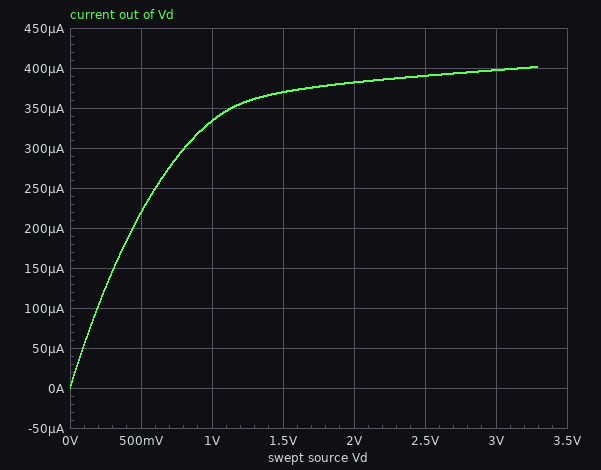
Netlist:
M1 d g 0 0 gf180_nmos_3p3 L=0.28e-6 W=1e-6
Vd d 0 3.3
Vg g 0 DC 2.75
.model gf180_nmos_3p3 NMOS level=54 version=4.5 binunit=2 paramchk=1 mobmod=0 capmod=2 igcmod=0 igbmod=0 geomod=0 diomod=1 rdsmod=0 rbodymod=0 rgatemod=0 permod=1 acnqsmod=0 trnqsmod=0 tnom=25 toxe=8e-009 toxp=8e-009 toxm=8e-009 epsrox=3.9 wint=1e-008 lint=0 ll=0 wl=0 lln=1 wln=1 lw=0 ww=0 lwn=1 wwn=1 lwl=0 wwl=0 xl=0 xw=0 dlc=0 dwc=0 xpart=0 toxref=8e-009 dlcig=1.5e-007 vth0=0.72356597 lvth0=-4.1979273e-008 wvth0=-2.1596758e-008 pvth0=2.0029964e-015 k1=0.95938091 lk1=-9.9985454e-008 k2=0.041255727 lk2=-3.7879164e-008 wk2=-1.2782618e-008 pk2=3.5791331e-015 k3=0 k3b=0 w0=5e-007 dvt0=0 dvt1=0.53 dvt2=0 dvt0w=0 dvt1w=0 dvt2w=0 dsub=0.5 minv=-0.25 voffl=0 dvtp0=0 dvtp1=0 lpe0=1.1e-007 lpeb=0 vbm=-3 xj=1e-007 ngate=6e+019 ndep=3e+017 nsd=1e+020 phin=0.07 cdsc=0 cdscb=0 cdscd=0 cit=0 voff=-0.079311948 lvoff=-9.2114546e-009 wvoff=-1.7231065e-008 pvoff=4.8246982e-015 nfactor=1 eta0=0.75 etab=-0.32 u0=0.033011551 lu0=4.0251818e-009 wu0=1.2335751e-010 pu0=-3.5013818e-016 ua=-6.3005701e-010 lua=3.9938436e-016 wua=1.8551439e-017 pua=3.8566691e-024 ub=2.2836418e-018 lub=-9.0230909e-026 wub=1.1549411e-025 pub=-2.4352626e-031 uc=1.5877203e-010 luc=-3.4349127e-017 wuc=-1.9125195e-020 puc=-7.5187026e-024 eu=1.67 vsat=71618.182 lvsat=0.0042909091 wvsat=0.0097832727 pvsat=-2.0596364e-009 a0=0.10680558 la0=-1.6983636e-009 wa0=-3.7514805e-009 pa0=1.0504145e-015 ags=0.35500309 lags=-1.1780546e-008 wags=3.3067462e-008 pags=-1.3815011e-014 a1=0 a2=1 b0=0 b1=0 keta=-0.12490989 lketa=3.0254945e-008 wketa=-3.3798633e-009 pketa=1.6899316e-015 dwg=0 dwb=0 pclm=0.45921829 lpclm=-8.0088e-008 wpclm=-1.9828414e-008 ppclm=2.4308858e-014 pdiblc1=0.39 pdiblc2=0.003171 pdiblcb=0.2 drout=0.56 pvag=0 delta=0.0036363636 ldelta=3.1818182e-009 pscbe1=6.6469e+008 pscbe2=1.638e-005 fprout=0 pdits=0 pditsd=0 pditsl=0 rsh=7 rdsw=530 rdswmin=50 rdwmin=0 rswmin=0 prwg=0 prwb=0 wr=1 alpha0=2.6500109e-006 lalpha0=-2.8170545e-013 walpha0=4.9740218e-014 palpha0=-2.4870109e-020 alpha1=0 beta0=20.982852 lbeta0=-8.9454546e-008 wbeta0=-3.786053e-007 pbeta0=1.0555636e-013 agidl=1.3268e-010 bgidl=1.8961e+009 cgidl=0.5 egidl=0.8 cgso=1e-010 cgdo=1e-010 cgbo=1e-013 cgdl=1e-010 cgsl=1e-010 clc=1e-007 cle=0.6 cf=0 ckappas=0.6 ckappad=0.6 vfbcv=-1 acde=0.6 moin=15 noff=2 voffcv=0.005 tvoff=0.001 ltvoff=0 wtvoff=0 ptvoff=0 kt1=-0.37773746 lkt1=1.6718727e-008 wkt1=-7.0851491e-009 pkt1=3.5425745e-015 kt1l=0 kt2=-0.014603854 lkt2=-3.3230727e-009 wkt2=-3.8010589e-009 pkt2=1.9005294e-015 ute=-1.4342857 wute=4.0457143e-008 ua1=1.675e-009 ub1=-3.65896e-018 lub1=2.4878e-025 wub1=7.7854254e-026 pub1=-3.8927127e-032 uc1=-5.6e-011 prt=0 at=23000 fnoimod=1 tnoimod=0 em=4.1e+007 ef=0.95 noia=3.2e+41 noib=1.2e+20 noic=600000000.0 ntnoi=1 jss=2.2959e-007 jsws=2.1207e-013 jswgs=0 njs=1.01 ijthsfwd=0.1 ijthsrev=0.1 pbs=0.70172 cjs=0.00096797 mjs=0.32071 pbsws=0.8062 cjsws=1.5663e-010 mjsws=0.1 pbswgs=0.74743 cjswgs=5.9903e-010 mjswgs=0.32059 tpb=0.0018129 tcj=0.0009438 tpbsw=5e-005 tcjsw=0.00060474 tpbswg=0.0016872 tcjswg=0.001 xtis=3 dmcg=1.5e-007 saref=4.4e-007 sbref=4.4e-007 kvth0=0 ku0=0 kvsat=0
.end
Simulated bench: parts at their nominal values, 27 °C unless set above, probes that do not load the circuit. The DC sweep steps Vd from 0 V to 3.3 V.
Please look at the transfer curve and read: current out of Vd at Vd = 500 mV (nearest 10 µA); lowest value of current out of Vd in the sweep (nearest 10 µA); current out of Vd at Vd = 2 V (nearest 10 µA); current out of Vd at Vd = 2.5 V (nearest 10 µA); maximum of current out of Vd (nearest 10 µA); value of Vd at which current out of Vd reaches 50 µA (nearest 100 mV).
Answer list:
220 µA
0 A
380 µA
390 µA
400 µA
100 mV
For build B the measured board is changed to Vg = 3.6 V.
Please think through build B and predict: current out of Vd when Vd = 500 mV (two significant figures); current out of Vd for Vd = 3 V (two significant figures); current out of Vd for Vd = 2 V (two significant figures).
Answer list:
270 µA
580 µA
560 µA
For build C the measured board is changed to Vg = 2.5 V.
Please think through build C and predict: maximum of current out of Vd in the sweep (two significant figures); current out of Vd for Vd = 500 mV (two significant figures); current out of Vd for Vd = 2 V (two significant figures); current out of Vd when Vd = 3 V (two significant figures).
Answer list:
350 µA
200 µA
330 µA
340 µA
